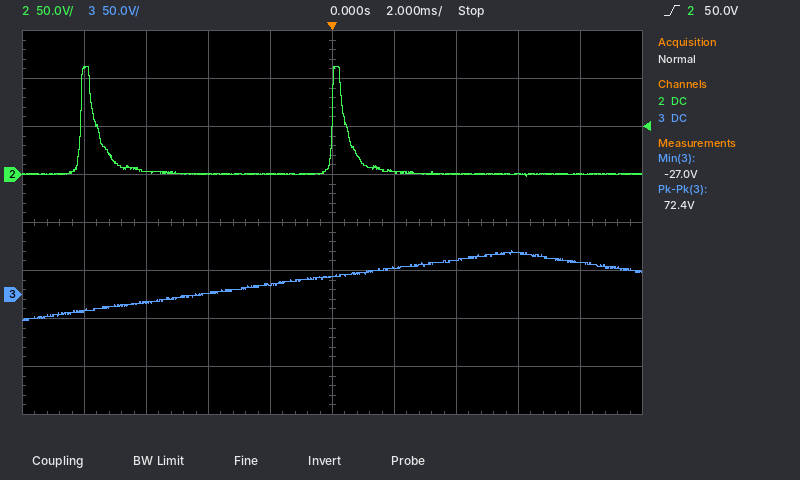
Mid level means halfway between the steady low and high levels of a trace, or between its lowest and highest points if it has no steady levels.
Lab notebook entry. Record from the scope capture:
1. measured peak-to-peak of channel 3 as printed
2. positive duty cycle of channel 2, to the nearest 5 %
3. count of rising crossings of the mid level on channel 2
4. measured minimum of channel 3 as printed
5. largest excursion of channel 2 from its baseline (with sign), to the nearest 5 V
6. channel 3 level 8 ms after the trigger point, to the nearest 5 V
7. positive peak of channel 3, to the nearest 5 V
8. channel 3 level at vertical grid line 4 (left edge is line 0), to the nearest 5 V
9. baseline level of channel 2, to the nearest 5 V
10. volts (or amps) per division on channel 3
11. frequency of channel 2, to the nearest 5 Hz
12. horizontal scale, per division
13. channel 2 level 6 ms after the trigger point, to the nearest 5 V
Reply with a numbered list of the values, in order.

1. 72.4 V
2. 5 %
3. 2
4. -27.0 V
5. +110 V
6. 35 V
7. 45 V
8. 10 V
9. 0 V
10. 50 V
11. 125 Hz
12. 2 ms
13. 0 V
